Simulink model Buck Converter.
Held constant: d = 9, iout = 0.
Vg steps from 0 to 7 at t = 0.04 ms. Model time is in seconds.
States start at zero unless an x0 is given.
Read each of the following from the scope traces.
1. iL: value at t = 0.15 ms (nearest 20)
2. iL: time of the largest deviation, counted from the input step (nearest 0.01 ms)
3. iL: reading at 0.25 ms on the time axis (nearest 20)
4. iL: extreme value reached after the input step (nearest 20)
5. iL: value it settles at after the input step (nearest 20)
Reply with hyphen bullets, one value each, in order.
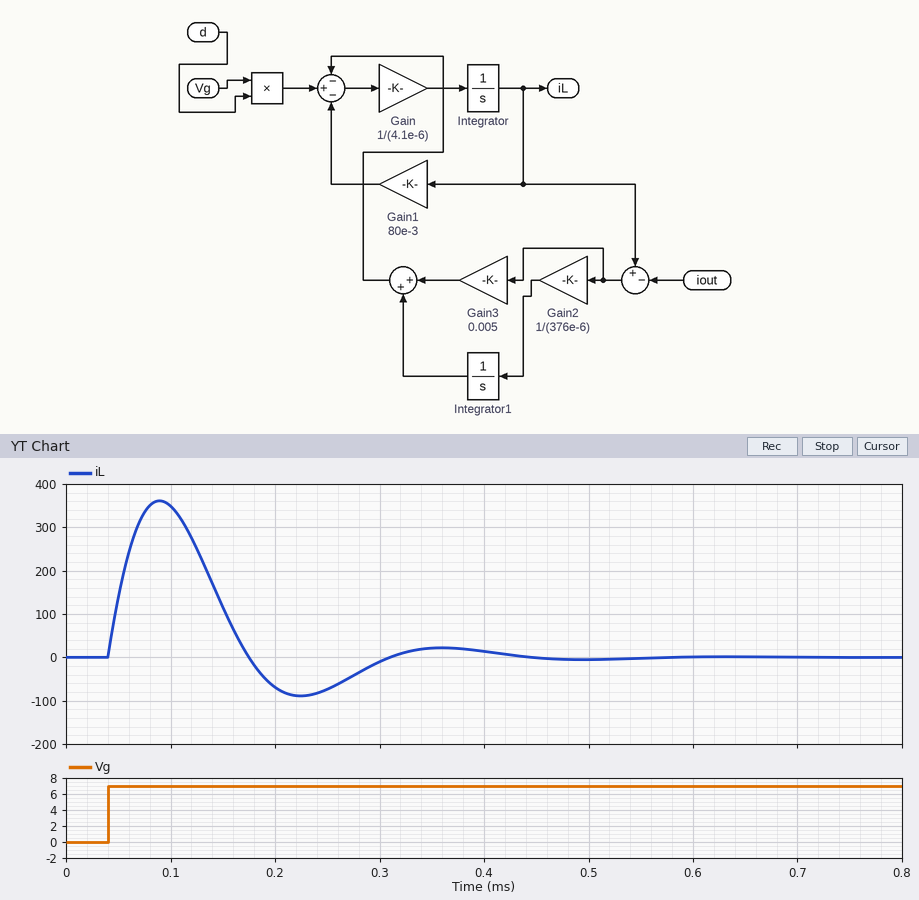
- 120
- 0.05 ms
- -80
- 360
- 0
